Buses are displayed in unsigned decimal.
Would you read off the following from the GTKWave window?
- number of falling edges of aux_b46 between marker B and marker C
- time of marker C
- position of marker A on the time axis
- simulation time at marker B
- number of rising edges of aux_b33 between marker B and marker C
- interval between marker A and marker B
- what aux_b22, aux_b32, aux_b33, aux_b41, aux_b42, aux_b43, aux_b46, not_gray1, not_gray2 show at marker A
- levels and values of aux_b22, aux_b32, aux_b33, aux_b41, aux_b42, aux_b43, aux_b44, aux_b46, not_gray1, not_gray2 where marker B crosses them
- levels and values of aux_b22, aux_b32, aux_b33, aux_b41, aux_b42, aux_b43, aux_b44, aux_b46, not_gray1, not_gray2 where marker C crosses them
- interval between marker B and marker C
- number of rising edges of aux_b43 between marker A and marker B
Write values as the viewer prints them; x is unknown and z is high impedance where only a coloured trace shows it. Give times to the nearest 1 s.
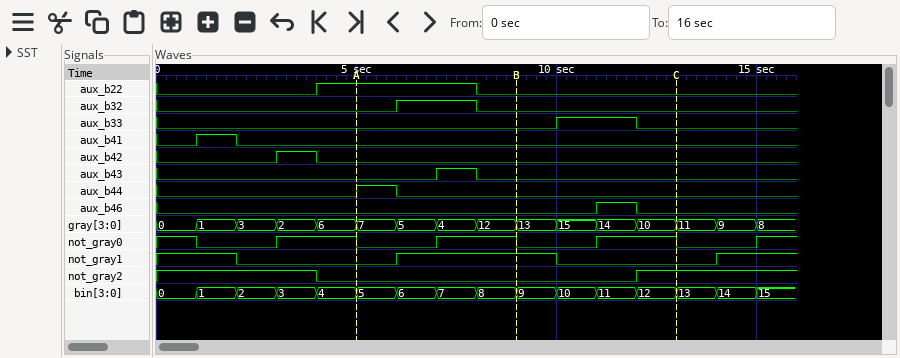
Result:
1
13 s
5 s
9 s
1
4 s
aux_b22=1, aux_b32=0, aux_b33=0, aux_b41=0, aux_b42=0, aux_b43=0, aux_b46=0, not_gray1=0, not_gray2=0
aux_b22=0, aux_b32=0, aux_b33=0, aux_b41=0, aux_b42=0, aux_b43=0, aux_b44=0, aux_b46=0, not_gray1=1, not_gray2=0
aux_b22=0, aux_b32=0, aux_b33=0, aux_b41=0, aux_b42=0, aux_b43=0, aux_b44=0, aux_b46=0, not_gray1=0, not_gray2=1
4 s
1
